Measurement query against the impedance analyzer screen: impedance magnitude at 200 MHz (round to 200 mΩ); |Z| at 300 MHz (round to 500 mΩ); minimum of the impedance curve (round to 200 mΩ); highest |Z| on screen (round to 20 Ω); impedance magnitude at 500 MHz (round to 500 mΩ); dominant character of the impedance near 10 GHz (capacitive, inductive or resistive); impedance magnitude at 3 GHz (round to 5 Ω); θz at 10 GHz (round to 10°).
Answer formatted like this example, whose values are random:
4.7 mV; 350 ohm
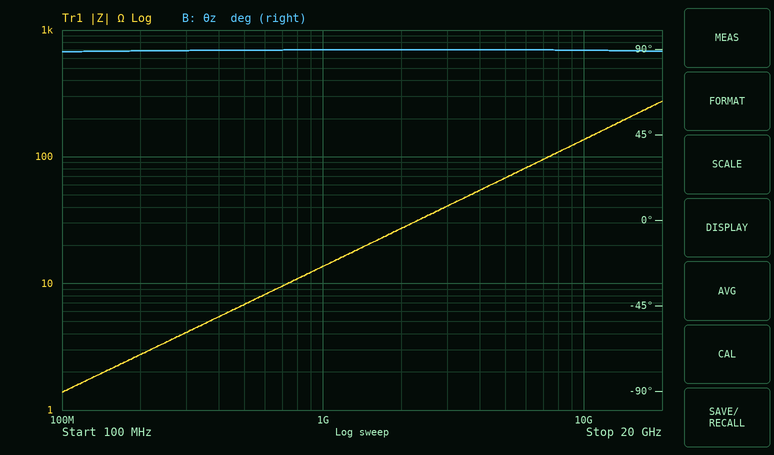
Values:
2.8 Ω; 4.0 Ω; 1.4 Ω; 280 Ω; 7.0 Ω; inductive; 40 Ω; 90°
